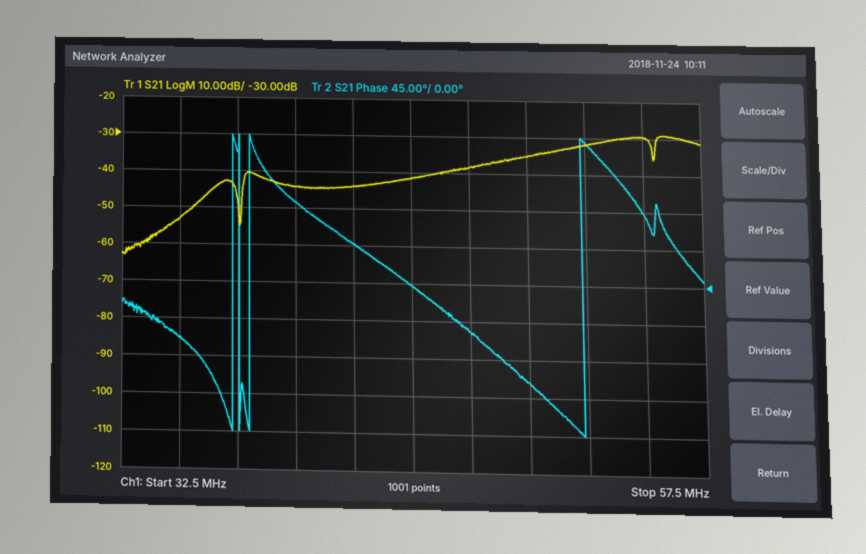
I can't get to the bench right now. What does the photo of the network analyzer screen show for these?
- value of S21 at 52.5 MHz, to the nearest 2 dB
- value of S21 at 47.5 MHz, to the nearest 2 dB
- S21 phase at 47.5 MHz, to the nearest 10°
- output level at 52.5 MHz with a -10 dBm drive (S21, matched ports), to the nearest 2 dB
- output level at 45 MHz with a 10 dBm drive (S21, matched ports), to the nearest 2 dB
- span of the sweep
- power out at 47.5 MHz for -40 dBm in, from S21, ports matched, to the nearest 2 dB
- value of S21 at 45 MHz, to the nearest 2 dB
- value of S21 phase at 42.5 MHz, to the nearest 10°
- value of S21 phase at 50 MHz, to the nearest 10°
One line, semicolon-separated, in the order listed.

-32 dB; -38 dB; -60°; -42 dBm; -32 dBm; 25 MHz; -78 dBm; -42 dB; 50°; -120°
